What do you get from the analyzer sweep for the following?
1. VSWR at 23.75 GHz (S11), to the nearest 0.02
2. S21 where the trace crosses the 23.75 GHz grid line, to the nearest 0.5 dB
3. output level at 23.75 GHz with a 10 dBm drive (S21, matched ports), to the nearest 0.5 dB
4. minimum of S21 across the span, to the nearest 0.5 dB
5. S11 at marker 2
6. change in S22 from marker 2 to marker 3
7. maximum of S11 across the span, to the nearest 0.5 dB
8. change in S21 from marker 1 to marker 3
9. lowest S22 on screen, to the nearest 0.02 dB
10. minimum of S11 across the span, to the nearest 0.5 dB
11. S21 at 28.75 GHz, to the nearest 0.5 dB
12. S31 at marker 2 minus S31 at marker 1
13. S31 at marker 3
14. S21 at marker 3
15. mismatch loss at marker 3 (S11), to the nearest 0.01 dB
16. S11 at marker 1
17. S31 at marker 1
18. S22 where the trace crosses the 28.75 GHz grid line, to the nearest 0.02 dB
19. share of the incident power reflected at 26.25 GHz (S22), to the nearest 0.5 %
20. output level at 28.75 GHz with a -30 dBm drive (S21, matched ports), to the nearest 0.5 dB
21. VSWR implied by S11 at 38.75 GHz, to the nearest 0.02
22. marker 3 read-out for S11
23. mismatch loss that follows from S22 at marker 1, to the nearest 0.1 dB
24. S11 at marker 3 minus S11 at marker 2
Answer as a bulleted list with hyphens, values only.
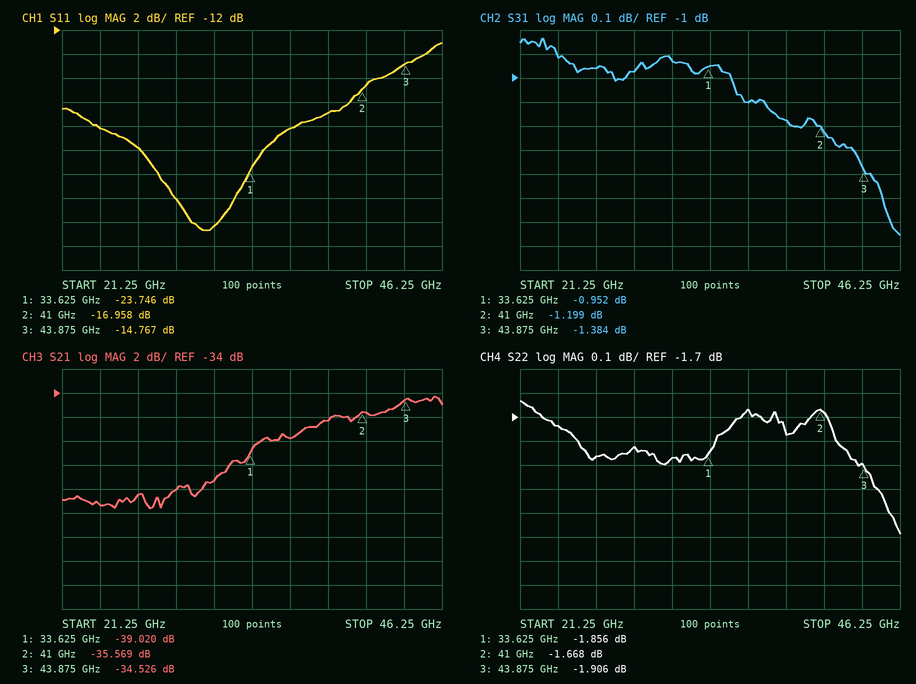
- 1.22
- -43.5 dB
- -33.5 dBm
- -43.5 dB
- -16.958 dB
- -0.238 dB
- -13.0 dB
- 4.494 dB
- -2.18 dB
- -28.5 dB
- -42.0 dB
- -0.247 dB
- -1.384 dB
- -34.526 dB
- 0.15 dB
- -23.746 dB
- -0.952 dB
- -1.82 dB
- 65.0 %
- -72.0 dBm
- 1.26
- -14.767 dB
- 4.6 dB
- 2.191 dB
